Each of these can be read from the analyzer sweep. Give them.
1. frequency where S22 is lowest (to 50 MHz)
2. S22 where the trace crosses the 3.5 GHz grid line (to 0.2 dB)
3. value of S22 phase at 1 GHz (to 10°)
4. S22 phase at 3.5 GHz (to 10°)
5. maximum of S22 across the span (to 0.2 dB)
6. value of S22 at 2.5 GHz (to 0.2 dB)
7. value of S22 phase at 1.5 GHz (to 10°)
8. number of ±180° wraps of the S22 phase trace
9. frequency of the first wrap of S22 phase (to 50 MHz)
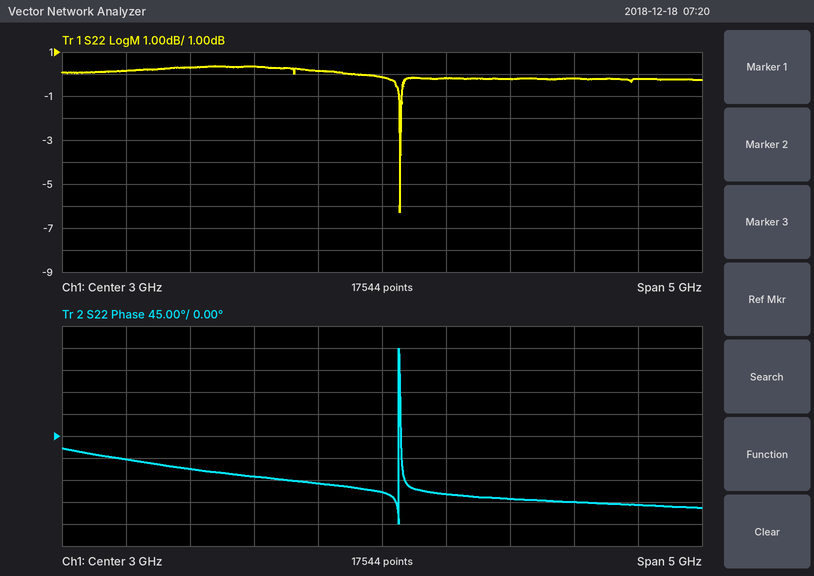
3.15 GHz
-0.2 dB
-50°
-120°
0.4 dB
0.2 dB
-70°
1
3.15 GHz
